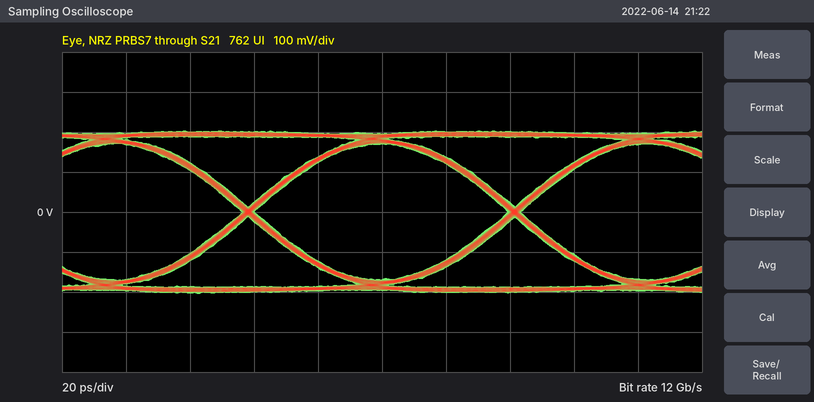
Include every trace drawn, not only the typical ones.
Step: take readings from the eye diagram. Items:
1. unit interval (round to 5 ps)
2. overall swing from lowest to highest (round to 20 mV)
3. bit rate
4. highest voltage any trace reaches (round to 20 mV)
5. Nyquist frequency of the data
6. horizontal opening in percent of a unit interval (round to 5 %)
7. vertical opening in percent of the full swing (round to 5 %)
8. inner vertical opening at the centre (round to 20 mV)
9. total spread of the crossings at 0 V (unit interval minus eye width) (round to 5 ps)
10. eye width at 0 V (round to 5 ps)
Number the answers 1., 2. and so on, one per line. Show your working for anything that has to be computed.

1. 85 ps
2. 400 mV
3. 12 Gb/s
4. 200 mV
5. 6 GHz
6. 80 ps / 85 ps ≈ 94.1 %, so 95 % to the nearest 5 %
7. 340 mV / 400 mV ≈ 85 %
8. 340 mV
9. 5 ps
10. 80 ps
